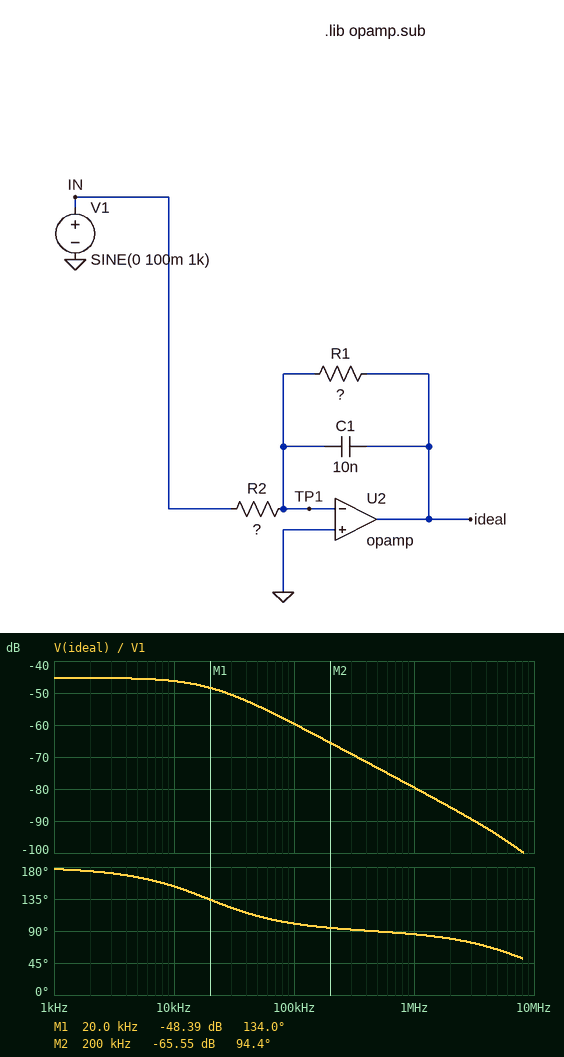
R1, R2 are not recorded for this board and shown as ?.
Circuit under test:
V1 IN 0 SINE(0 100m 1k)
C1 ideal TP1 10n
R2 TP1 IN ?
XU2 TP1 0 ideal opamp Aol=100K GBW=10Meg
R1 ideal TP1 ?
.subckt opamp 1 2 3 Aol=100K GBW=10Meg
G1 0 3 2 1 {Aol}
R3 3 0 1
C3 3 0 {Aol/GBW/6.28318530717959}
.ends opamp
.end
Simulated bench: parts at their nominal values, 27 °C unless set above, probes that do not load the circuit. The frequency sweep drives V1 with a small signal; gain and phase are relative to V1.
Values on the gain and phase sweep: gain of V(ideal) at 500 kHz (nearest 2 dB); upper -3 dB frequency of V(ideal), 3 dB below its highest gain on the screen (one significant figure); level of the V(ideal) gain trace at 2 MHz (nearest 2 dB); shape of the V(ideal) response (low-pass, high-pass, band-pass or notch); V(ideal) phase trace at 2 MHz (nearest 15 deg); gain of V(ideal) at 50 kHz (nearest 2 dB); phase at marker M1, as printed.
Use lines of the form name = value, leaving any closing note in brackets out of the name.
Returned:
gain of V(ideal) at 500 kHz = -74 dB
upper -3 dB frequency of V(ideal), 3 dB below its highest gain on the screen = 20 kHz
level of the V(ideal) gain trace at 2 MHz = -86 dB
shape of the V(ideal) response = low-pass
V(ideal) phase trace at 2 MHz = 75 deg
gain of V(ideal) at 50 kHz = -54 dB
phase at marker M1, as printed = 134.0 deg
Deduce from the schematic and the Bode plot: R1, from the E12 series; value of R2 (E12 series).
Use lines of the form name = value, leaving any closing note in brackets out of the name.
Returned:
R1, from the E12 series = 820 Ω
value of R2 = 150 kΩ
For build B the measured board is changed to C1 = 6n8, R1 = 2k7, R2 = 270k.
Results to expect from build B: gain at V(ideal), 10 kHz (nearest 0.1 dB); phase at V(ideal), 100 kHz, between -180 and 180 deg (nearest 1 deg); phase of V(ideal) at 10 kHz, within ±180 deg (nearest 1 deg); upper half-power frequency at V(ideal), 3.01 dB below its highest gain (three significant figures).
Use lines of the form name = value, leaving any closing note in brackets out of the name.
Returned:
gain at V(ideal), 10 kHz = -43.7 dB
phase at V(ideal), 100 kHz, between -180 and 180 deg = 94 deg
phase of V(ideal) at 10 kHz, within ±180 deg = 131 deg
upper half-power frequency at V(ideal), 3.01 dB below its highest gain = 8.67 kHz
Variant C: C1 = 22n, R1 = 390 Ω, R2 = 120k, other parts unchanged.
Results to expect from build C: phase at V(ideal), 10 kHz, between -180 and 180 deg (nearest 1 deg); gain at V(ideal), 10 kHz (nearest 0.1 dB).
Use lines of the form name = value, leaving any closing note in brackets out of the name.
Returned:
phase at V(ideal), 10 kHz, between -180 and 180 deg = 152 deg
gain at V(ideal), 10 kHz = -50.9 dB
